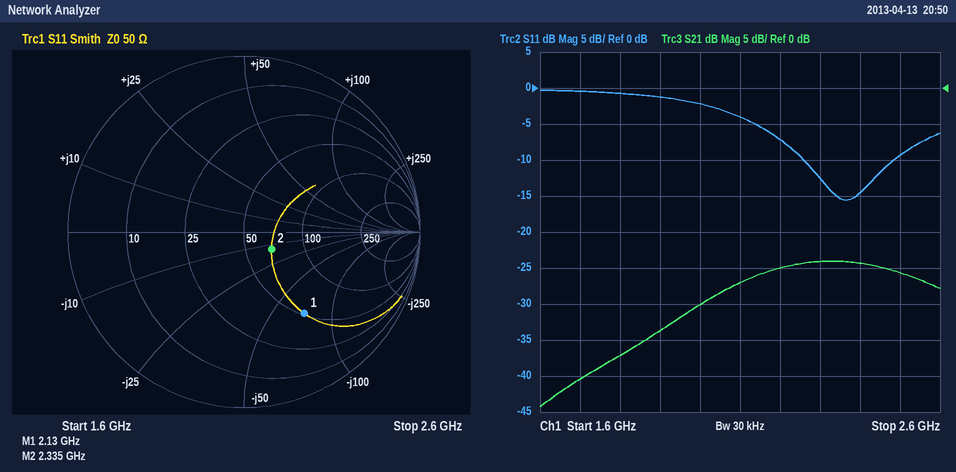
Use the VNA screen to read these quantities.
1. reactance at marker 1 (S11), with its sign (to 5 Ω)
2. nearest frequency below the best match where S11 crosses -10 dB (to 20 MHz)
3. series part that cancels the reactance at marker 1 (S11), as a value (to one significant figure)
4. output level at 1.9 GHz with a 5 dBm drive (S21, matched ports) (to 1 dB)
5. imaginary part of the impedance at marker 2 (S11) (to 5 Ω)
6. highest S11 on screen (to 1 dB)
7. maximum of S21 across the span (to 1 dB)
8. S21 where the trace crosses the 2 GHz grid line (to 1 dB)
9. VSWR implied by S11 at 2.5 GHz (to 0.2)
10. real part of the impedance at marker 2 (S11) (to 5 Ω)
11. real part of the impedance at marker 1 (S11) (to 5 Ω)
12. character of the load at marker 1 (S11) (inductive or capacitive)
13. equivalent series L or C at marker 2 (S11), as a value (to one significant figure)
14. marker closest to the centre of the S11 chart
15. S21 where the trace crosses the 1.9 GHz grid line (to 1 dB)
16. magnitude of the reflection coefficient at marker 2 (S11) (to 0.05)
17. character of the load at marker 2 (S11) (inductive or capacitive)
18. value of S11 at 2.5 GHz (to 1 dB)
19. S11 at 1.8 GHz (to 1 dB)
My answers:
-70 Ω
2.26 GHz
5 nH
-29 dBm
-15 Ω
0 dB
-24 dB
-30 dB
2.0
65 Ω
50 Ω
capacitive
5 pF
marker 2
-34 dB
0.20
capacitive
-9 dB
-1 dB
